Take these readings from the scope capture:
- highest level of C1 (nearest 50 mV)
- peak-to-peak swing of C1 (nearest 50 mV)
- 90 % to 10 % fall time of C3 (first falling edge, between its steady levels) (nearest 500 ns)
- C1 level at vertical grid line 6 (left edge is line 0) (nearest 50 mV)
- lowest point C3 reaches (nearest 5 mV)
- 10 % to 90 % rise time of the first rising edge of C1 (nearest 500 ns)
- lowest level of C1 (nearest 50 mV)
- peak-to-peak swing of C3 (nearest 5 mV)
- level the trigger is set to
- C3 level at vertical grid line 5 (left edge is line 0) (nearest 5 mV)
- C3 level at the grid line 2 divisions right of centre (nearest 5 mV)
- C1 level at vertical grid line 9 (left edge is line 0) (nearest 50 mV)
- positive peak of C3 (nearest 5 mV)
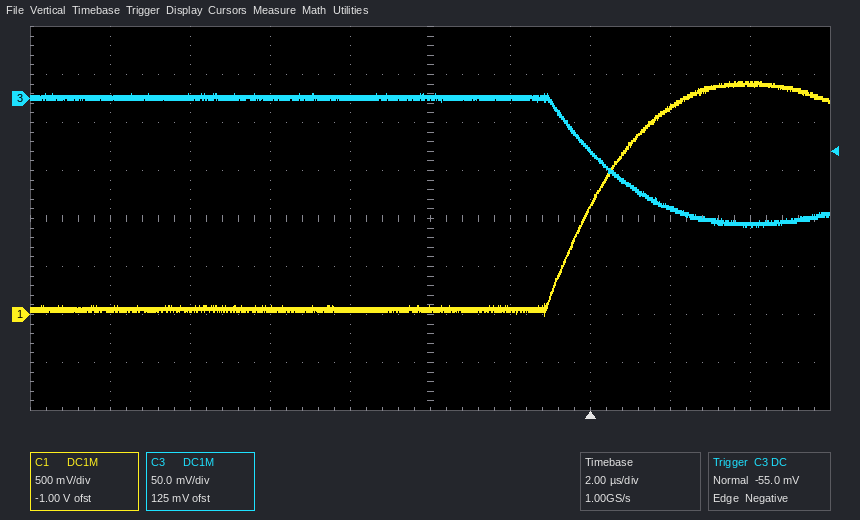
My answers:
2.45 V
2.45 V
3.0 µs
50 mV
-135 mV
3.0 µs
0 mV
140 mV
-55.0 mV
0 mV
-55 mV
2.40 V
5 mV
